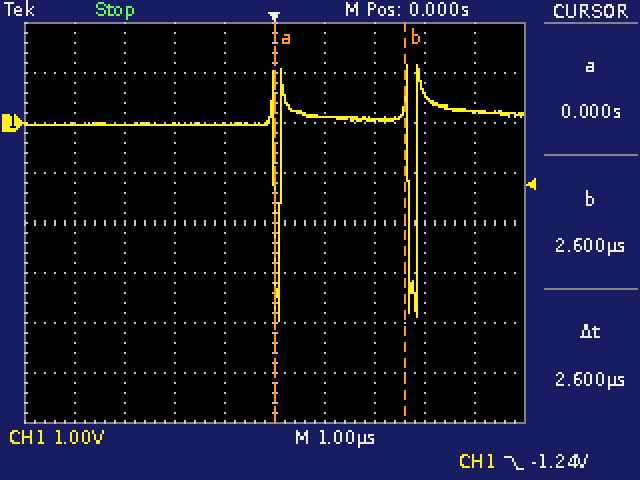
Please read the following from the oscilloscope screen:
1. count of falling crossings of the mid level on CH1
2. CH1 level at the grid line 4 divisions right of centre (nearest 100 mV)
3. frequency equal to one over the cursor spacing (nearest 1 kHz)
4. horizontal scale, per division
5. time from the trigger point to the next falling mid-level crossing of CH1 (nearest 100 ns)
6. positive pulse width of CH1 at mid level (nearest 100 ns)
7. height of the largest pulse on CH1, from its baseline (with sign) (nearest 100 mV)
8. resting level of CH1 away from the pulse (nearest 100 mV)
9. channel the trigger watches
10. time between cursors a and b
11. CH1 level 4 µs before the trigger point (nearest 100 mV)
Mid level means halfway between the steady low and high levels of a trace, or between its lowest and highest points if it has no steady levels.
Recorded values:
2
200 mV
385 kHz
1 µs
2.7 µs
2.6 µs
-3.9 V
0.0 V
CH1
2.6 µs
0.0 V
